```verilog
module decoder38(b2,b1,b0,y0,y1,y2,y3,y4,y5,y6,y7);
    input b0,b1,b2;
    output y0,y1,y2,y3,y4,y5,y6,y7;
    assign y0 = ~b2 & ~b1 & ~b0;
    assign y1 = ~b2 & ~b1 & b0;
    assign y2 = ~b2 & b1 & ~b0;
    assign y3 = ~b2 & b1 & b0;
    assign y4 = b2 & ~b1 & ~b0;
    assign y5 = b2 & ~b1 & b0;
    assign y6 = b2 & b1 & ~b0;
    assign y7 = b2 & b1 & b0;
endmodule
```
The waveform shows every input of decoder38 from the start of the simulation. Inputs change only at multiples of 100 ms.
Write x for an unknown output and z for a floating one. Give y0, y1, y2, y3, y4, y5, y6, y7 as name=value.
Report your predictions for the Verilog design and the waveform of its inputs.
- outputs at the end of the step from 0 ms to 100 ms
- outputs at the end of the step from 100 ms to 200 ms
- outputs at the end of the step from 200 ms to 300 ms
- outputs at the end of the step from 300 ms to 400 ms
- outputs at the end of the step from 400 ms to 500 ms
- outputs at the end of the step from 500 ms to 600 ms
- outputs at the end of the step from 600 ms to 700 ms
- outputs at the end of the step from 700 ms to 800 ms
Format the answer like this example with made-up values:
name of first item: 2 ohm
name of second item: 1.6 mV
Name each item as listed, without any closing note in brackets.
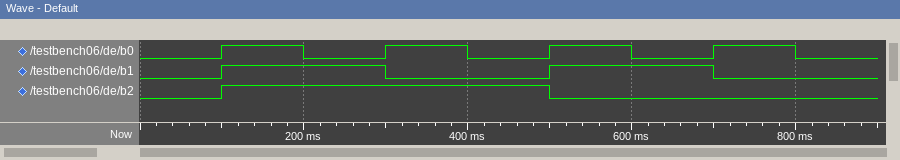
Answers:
outputs at the end of the step from 0 ms to 100 ms: y0=1, y1=0, y2=0, y3=0, y4=0, y5=0, y6=0, y7=0
outputs at the end of the step from 100 ms to 200 ms: y0=0, y1=0, y2=0, y3=0, y4=0, y5=0, y6=0, y7=1
outputs at the end of the step from 200 ms to 300 ms: y0=0, y1=0, y2=0, y3=0, y4=0, y5=0, y6=1, y7=0
outputs at the end of the step from 300 ms to 400 ms: y0=0, y1=0, y2=0, y3=0, y4=0, y5=1, y6=0, y7=0
outputs at the end of the step from 400 ms to 500 ms: y0=0, y1=0, y2=0, y3=0, y4=1, y5=0, y6=0, y7=0
outputs at the end of the step from 500 ms to 600 ms: y0=0, y1=0, y2=0, y3=1, y4=0, y5=0, y6=0, y7=0
outputs at the end of the step from 600 ms to 700 ms: y0=0, y1=0, y2=1, y3=0, y4=0, y5=0, y6=0, y7=0
outputs at the end of the step from 700 ms to 800 ms: y0=0, y1=1, y2=0, y3=0, y4=0, y5=0, y6=0, y7=0
